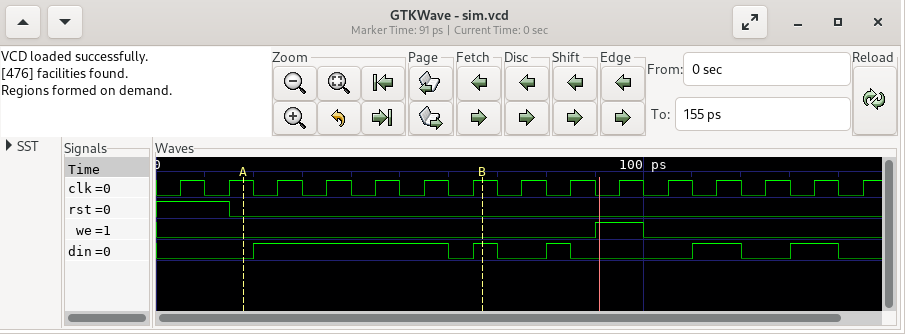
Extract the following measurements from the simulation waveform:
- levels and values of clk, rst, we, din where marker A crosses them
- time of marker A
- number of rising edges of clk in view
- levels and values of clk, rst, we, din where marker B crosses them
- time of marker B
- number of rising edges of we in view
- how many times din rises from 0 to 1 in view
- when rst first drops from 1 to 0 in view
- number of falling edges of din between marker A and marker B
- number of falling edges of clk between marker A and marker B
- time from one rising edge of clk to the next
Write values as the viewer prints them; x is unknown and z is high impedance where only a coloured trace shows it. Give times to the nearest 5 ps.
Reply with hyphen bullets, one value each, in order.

- clk=1, rst=0, we=0, din=0
- 20 ps
- 15
- clk=1, rst=0, we=0, din=1
- 65 ps
- 1
- 5
- 15 ps
- 1
- 5
- 10 ps
